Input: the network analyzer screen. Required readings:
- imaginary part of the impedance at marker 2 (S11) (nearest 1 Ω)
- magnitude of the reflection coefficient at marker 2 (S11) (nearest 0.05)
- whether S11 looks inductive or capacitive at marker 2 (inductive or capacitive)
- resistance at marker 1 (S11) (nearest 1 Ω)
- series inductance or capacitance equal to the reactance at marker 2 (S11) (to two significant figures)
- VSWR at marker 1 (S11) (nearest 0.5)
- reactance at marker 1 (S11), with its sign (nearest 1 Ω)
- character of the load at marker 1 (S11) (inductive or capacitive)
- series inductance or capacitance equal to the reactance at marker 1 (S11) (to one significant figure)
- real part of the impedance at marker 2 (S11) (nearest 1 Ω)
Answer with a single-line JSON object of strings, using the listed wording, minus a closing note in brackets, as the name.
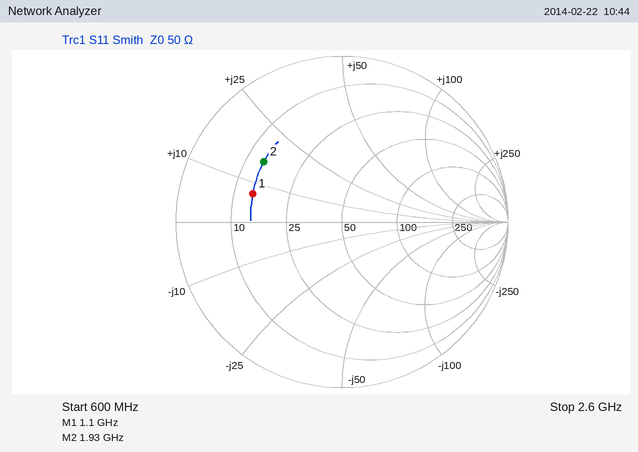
{"imaginary part of the impedance at marker 2 (S11)": "+16 Ω", "magnitude of the reflection coefficient at marker 2 (S11)": "0.60", "whether S11 looks inductive or capacitive at marker 2": "inductive", "resistance at marker 1 (S11)": "14 Ω", "series inductance or capacitance equal to the reactance at marker 2 (S11)": "1.3 nH", "VSWR at marker 1 (S11)": "3.5", "reactance at marker 1 (S11), with its sign": "+7 Ω", "character of the load at marker 1 (S11)": "inductive", "series inductance or capacitance equal to the reactance at marker 1 (S11)": "1 nH", "real part of the impedance at marker 2 (S11)": "14 Ω"}
